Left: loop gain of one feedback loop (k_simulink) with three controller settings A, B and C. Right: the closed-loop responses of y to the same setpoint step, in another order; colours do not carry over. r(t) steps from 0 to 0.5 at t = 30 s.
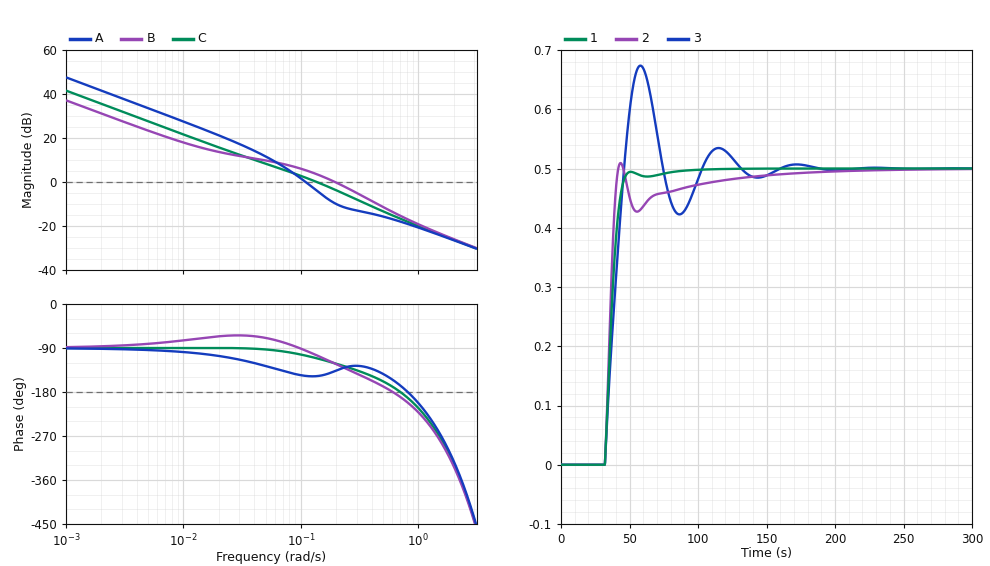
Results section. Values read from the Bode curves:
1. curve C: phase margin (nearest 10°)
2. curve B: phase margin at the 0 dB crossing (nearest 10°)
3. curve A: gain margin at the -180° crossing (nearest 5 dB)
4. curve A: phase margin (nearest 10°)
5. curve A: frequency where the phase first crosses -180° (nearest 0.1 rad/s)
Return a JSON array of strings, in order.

["70°", "60°", "20 dB", "30°", "0.8 rad/s"]
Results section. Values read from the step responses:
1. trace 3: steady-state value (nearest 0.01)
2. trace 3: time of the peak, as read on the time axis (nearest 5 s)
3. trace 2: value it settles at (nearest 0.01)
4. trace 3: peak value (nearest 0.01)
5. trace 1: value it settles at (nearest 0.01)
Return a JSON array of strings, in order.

["0.50", "60 s", "0.50", "0.67", "0.50"]
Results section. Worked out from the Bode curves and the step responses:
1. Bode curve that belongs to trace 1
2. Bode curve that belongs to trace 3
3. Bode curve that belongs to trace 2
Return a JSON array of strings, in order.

["C", "A", "B"]
